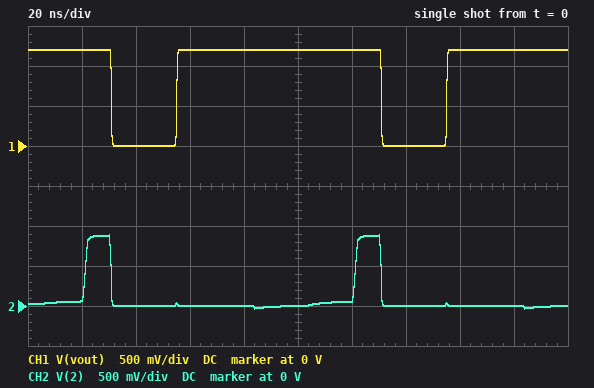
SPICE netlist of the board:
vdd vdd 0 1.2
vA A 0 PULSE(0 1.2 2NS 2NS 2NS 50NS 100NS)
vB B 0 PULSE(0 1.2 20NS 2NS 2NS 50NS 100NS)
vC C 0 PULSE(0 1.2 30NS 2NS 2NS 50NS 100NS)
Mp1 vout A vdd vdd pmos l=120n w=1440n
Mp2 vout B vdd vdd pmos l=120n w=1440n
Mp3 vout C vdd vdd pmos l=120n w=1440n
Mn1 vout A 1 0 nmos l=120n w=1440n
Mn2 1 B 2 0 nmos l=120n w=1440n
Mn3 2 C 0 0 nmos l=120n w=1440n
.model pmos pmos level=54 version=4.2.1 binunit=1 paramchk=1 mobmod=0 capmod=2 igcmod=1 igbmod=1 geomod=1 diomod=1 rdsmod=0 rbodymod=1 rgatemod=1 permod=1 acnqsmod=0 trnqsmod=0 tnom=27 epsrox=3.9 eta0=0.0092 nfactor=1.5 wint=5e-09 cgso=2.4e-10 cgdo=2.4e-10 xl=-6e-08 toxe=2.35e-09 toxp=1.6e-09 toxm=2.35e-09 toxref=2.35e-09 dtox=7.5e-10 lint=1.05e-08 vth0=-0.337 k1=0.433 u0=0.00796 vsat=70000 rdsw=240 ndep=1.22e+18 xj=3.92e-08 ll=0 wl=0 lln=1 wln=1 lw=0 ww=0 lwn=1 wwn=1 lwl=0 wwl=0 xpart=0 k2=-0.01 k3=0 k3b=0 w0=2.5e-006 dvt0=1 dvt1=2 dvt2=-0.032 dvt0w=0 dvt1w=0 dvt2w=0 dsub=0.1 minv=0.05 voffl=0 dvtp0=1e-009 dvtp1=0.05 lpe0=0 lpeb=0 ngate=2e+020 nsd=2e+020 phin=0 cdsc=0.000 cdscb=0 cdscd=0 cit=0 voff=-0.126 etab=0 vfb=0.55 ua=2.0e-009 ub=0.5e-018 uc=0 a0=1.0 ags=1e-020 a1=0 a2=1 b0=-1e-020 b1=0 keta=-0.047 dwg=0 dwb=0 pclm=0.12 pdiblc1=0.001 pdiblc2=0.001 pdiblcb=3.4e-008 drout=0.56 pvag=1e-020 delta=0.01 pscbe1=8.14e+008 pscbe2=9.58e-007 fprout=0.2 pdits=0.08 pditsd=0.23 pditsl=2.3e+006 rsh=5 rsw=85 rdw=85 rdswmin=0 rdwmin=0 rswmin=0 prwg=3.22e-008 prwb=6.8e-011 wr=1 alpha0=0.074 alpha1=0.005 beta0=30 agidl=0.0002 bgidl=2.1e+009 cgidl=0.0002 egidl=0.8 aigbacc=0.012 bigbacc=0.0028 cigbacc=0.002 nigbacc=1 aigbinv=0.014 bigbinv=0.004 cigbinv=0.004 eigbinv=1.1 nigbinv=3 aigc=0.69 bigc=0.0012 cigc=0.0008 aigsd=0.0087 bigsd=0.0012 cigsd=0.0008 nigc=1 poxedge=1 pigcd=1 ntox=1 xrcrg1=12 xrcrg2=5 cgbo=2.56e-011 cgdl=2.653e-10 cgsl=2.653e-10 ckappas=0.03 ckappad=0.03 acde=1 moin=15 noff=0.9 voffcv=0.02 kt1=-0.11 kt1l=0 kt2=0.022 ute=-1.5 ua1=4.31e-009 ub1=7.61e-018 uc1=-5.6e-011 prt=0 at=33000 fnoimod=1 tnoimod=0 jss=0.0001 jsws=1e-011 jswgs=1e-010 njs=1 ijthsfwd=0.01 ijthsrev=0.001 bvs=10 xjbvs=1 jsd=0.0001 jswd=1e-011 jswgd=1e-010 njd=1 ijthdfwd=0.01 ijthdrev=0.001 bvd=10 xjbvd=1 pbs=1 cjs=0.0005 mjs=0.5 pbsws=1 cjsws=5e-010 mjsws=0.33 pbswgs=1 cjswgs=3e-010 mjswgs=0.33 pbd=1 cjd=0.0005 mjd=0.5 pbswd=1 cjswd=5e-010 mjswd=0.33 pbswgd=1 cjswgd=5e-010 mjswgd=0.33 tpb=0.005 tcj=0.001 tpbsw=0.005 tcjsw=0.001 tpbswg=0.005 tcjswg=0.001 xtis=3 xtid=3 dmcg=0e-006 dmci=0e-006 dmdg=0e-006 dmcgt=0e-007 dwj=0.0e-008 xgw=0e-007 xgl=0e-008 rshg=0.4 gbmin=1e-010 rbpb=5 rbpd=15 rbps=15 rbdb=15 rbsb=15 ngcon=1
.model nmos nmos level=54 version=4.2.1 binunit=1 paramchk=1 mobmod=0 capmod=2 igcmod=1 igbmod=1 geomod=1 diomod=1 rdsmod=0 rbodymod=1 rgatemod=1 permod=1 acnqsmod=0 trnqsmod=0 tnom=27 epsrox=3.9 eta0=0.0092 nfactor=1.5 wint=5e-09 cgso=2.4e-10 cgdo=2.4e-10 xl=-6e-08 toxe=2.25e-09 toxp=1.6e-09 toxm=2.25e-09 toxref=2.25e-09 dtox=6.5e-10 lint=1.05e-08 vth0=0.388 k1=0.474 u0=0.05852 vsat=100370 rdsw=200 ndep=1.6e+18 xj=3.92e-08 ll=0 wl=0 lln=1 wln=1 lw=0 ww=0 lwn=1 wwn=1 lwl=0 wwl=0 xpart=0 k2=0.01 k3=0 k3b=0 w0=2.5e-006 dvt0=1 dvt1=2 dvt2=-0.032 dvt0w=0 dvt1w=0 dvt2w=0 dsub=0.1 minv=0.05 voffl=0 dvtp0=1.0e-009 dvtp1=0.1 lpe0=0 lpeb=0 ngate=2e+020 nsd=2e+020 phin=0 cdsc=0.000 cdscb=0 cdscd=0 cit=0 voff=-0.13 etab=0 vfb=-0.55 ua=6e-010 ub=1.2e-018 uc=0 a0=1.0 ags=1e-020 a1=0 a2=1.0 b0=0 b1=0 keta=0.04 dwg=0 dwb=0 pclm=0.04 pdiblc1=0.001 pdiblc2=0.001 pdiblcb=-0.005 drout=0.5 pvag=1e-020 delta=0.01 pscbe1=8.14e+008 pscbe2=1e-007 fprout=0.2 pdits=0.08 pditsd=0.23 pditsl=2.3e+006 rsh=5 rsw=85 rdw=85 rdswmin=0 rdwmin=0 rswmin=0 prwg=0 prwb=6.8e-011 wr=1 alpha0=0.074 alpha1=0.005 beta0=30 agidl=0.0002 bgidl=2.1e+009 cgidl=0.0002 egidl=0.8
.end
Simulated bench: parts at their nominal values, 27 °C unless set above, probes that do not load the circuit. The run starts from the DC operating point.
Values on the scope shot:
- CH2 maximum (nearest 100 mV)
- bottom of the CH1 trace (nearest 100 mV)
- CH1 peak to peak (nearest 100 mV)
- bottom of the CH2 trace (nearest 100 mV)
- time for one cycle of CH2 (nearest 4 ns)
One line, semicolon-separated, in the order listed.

900 mV; 0 V; 1.2 V; 0 V; 100 ns
